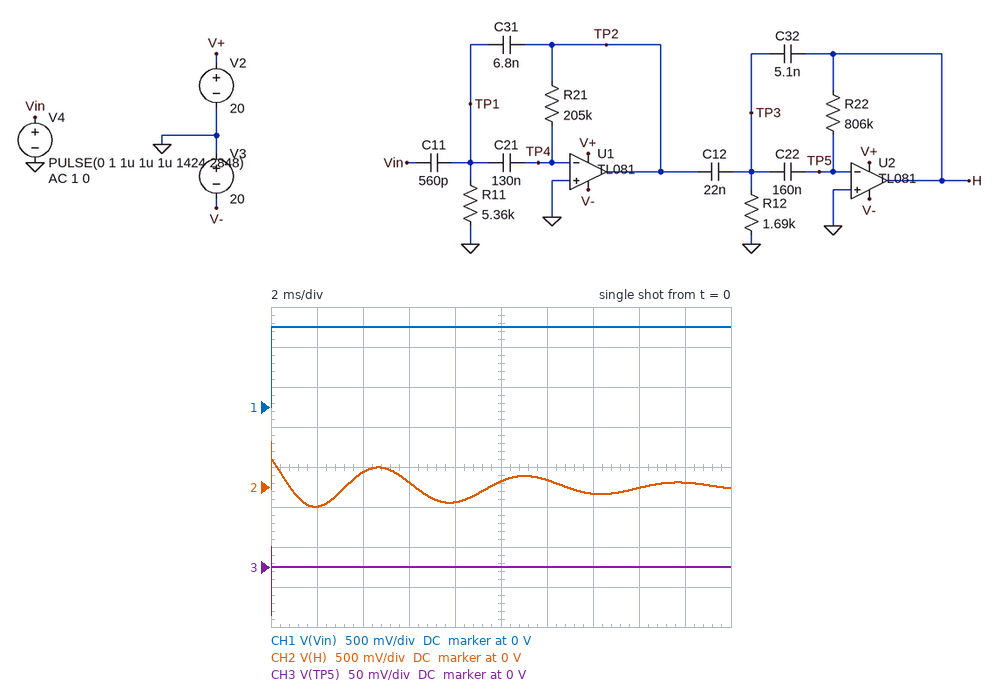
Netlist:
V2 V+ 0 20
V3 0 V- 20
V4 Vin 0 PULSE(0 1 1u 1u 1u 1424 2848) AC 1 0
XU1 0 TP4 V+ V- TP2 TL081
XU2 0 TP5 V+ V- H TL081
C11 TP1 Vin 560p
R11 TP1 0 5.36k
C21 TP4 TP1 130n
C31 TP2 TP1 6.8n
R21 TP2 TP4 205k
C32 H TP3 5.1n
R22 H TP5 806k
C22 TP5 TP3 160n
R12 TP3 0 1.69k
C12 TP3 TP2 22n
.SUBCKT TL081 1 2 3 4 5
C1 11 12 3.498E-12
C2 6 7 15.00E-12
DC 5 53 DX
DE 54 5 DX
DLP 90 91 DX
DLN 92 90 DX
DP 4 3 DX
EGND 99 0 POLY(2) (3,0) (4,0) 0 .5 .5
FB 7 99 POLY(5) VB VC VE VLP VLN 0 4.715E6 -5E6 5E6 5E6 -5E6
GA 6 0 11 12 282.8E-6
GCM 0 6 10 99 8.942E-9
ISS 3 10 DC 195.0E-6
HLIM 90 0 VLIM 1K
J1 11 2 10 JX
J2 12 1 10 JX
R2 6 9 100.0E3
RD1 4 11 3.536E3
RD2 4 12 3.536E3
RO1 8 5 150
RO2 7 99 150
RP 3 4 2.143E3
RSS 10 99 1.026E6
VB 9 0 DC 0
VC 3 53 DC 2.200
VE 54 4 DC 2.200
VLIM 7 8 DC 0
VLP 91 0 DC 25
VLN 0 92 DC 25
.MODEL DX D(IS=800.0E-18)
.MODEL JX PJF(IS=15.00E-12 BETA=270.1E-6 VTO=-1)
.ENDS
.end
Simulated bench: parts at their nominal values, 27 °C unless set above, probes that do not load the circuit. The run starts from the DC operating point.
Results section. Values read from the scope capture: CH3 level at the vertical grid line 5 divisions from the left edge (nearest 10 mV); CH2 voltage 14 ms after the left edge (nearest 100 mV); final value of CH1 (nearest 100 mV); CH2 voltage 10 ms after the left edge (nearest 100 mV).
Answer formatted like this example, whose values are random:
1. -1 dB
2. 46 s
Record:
1. 0 V
2. -100 mV
3. 1.0 V
4. 100 mV
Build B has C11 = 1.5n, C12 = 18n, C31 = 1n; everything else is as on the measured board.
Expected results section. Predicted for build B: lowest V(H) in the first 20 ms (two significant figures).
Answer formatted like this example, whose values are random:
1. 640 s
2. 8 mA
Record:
1. -1.2 V
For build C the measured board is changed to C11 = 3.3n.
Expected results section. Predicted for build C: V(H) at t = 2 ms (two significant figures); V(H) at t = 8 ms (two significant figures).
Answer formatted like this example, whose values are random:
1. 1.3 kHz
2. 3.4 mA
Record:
1. -1.4 V
2. -1.1 V
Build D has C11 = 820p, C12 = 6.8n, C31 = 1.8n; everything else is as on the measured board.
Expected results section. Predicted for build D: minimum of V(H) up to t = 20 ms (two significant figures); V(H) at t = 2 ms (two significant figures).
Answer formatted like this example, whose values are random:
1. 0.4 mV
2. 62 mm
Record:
1. -210 mV
2. -57 mV
